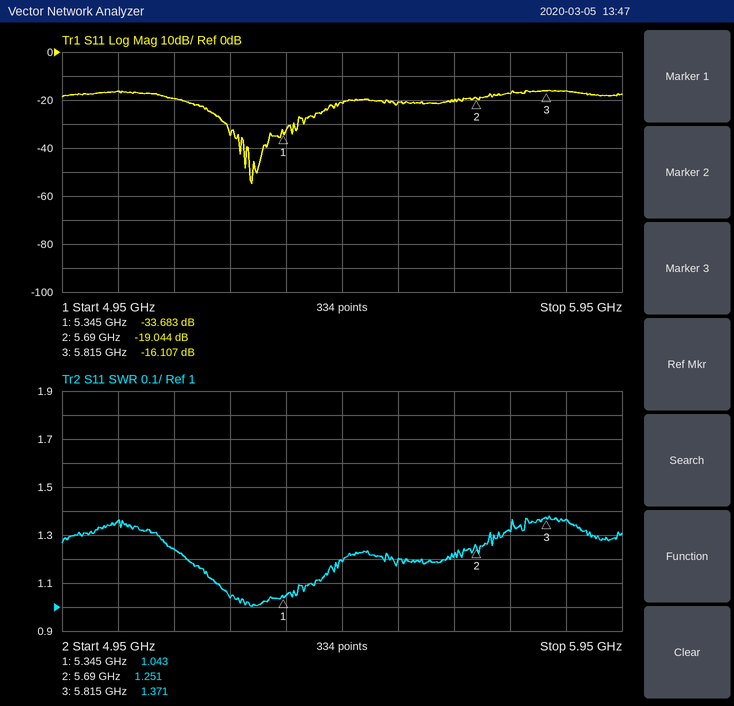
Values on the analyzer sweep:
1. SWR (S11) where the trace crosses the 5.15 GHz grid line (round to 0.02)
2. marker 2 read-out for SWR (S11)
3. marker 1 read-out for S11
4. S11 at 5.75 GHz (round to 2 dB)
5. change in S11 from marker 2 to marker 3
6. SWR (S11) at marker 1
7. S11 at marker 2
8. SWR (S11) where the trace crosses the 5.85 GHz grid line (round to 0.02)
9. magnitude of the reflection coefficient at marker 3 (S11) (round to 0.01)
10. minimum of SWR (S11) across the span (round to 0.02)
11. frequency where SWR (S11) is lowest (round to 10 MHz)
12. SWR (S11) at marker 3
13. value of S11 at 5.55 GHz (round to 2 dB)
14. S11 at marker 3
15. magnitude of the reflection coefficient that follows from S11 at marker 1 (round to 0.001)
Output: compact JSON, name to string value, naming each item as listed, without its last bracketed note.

{"SWR (S11) where the trace crosses the 5.15 GHz grid line": "1.24", "marker 2 read-out for SWR": "1.251", "marker 1 read-out for S11": "-33.683 dB", "S11 at 5.75 GHz": "-18 dB", "change in S11 from marker 2 to marker 3": "2.937 dB", "SWR (S11) at marker 1": "1.043", "S11 at marker 2": "-19.044 dB", "SWR (S11) where the trace crosses the 5.85 GHz grid line": "1.36", "magnitude of the reflection coefficient at marker 3 (S11)": "0.16", "minimum of SWR (S11) across the span": "1.00", "frequency where SWR (S11) is lowest": "5.29 GHz", "SWR (S11) at marker 3": "1.371", "value of S11 at 5.55 GHz": "-20 dB", "S11 at marker 3": "-16.107 dB", "magnitude of the reflection coefficient that follows from S11 at marker 1": "0.021"}
